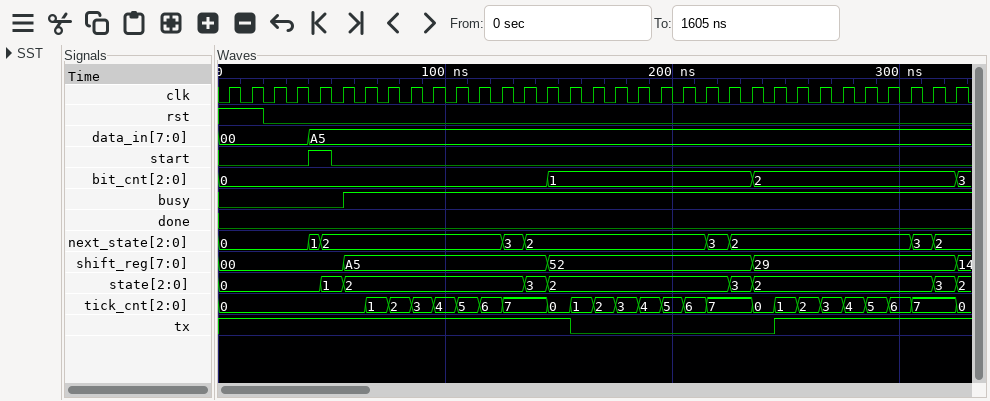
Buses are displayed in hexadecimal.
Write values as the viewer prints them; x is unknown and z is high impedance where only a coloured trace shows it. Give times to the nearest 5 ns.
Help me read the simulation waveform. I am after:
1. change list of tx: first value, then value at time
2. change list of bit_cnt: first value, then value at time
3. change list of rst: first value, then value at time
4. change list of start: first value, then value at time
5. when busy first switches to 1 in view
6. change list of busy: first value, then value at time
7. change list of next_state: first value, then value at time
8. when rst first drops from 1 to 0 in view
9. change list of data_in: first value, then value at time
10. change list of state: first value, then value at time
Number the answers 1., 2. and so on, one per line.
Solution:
1. 1, 0 at 155 ns, 1 at 245 ns
2. 0, 1 at 145 ns, 2 at 235 ns, 3 at 325 ns
3. 1, 0 at 20 ns
4. 0, 1 at 40 ns, 0 at 50 ns
5. 55 ns
6. 0, 1 at 55 ns
7. 0, 1 at 40 ns, 2 at 45 ns, 3 at 125 ns, 2 at 135 ns, 3 at 215 ns, 2 at 225 ns, 3 at 305 ns, 2 at 315 ns
8. 20 ns
9. 00, A5 at 40 ns
10. 0, 1 at 45 ns, 2 at 55 ns, 3 at 135 ns, 2 at 145 ns, 3 at 225 ns, 2 at 235 ns, 3 at 315 ns, 2 at 325 ns
